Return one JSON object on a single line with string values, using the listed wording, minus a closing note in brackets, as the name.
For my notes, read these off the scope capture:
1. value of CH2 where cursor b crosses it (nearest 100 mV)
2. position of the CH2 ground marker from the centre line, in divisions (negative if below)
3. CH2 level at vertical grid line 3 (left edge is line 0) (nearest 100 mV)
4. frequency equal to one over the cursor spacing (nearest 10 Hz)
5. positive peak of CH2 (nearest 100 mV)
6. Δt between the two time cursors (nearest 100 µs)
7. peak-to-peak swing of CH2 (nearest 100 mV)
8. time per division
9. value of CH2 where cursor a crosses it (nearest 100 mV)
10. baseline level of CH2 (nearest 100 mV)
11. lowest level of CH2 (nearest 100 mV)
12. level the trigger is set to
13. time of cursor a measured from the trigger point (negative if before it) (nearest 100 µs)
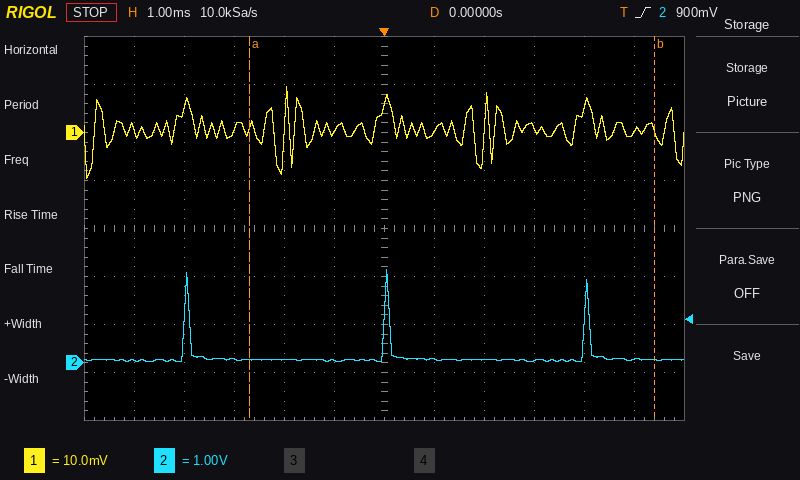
{"value of CH2 where cursor b crosses it": "100 mV", "position of the CH2 ground marker from the centre line, in divisions": "-2.8 div", "CH2 level at vertical grid line 3 (left edge is line 0)": "100 mV", "frequency equal to one over the cursor spacing": "120 Hz", "positive peak of CH2": "1.9 V", "Δt between the two time cursors": "8.1 ms", "peak-to-peak swing of CH2": "1.9 V", "time per division": "1 ms", "value of CH2 where cursor a crosses it": "100 mV", "baseline level of CH2": "100 mV", "lowest level of CH2": "0.0 V", "level the trigger is set to": "900 mV", "time of cursor a measured from the trigger point (negative if before it)": "-2.7 ms"}
